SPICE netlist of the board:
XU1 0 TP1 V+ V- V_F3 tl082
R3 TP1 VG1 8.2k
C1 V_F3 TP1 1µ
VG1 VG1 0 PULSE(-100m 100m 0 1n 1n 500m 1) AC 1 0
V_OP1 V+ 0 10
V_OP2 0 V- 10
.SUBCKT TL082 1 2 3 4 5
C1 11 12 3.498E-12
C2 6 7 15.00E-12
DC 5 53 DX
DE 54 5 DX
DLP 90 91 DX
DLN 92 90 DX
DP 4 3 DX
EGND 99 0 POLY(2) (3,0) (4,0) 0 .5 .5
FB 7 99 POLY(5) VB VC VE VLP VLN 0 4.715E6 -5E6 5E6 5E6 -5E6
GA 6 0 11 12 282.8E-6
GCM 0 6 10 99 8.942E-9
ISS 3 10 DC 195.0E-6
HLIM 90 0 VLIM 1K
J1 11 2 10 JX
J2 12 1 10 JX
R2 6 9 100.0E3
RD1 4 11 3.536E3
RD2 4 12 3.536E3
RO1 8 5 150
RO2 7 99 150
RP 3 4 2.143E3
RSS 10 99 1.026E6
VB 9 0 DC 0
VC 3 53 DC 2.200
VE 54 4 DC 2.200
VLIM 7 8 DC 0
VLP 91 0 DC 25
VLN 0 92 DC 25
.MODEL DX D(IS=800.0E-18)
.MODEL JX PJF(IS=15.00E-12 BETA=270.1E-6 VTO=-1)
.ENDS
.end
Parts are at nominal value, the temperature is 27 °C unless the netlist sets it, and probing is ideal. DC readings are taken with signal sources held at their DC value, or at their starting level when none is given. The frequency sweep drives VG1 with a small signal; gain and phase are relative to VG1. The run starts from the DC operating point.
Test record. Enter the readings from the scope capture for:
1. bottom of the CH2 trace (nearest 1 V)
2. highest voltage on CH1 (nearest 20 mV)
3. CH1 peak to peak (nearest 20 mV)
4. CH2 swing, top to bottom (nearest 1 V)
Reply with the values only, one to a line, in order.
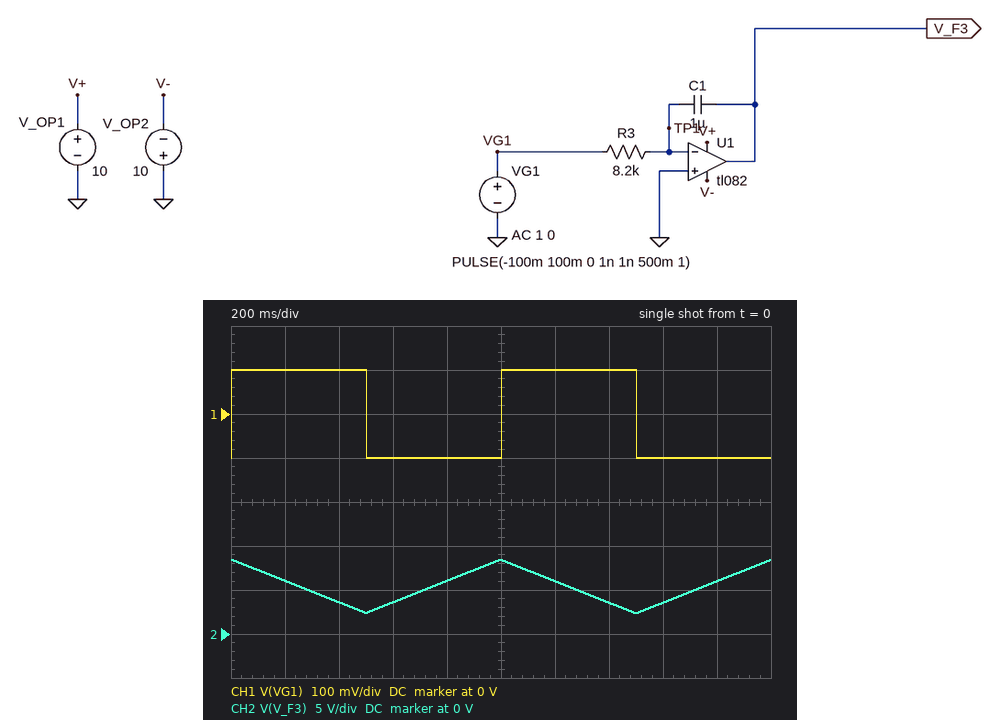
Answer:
2 V
100 mV
200 mV
6 V
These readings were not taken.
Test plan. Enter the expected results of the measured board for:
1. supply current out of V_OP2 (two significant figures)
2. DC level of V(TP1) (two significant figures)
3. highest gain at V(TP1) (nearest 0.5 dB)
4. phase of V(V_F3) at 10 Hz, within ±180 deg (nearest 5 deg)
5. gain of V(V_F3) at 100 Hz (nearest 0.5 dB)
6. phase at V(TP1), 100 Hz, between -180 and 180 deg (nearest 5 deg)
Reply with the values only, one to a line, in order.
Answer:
9.5 mA
-100 mV
0 dB
145 deg
-28.0 dB
-80 deg
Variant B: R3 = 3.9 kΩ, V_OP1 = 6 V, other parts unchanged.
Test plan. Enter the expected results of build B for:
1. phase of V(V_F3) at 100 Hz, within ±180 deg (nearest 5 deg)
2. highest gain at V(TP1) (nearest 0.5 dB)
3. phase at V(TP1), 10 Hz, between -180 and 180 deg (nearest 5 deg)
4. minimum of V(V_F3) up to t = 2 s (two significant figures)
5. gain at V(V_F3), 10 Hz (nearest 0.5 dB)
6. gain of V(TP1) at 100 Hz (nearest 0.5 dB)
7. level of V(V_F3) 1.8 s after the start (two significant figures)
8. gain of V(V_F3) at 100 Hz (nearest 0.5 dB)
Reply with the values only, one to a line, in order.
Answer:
110 deg
0 dB
-15 deg
-8.4 V
-12.0 dB
-10.0 dB
-700 mV
-22.0 dB
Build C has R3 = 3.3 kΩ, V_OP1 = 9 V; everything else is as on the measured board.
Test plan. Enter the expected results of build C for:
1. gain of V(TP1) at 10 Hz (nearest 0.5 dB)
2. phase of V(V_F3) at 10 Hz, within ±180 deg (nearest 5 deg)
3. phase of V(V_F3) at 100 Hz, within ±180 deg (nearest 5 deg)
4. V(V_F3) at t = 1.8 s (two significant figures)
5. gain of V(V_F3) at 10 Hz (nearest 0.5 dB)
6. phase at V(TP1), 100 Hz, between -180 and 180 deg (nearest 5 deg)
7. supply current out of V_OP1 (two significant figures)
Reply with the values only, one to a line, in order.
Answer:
-0.5 dB
165 deg
110 deg
1.4 V
-12.0 dB
-70 deg
9.0 mA
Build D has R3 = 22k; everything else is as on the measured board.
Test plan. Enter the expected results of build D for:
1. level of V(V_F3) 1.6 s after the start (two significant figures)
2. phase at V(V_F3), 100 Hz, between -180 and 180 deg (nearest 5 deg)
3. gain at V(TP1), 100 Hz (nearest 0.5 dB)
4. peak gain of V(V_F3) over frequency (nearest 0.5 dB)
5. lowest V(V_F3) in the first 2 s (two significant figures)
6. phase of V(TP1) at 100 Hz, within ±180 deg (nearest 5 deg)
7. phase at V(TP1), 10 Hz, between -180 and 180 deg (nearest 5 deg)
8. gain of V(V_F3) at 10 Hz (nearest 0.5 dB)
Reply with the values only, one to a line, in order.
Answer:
6.6 V
95 deg
-25.0 dB
-12.0 dB
6.2 V
-85 deg
-60 deg
-18.0 dB
